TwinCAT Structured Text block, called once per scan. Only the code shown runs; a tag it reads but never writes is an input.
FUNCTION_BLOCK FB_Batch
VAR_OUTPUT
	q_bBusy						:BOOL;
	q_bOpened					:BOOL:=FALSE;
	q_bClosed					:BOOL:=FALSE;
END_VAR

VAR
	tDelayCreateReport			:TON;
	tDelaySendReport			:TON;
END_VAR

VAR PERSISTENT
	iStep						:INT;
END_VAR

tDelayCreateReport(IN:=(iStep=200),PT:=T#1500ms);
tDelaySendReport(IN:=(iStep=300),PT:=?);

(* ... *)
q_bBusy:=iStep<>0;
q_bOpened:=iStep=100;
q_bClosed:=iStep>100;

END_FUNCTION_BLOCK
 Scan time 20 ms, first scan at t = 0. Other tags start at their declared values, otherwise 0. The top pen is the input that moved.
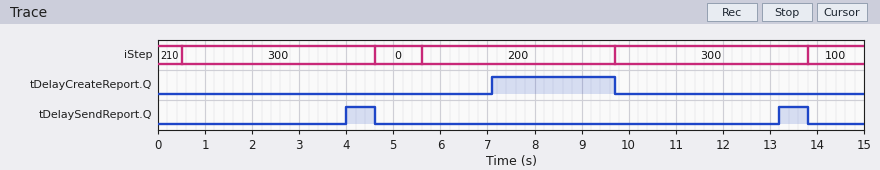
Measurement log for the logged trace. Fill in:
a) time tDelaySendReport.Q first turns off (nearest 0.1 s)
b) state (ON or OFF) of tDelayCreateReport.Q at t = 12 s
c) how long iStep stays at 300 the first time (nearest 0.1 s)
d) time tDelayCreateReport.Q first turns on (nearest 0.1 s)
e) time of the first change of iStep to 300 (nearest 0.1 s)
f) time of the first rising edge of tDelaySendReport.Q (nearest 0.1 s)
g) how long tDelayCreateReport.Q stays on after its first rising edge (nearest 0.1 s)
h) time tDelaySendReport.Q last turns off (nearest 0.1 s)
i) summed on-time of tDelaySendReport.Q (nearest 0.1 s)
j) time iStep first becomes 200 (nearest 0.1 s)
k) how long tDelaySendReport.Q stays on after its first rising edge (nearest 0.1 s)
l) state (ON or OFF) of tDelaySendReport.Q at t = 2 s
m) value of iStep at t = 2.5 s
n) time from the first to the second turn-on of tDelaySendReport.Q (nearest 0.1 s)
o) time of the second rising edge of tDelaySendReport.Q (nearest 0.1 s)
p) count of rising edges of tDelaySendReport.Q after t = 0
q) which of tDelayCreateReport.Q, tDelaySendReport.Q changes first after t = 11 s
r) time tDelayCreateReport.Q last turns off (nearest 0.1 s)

4.6 s
OFF
4.1 s
7.1 s
0.5 s
4.0 s
2.6 s
13.8 s
1.2 s
5.6 s
0.6 s
OFF
300
9.2 s
13.2 s
2
tDelaySendReport.Q
9.7 s
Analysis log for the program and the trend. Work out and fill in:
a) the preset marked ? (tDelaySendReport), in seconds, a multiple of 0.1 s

3.5 s
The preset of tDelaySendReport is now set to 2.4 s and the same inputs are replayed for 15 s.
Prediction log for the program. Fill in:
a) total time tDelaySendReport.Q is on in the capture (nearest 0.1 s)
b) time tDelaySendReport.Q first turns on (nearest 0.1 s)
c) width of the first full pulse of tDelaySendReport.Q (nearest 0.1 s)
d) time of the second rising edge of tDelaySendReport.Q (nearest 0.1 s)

3.4 s
2.9 s
1.7 s
12.1 s
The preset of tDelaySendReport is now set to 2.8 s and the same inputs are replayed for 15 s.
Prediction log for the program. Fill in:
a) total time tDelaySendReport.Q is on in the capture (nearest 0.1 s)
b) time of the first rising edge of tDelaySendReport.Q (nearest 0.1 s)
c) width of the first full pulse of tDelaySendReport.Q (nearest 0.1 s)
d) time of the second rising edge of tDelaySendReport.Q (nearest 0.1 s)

2.6 s
3.3 s
1.3 s
12.5 s
